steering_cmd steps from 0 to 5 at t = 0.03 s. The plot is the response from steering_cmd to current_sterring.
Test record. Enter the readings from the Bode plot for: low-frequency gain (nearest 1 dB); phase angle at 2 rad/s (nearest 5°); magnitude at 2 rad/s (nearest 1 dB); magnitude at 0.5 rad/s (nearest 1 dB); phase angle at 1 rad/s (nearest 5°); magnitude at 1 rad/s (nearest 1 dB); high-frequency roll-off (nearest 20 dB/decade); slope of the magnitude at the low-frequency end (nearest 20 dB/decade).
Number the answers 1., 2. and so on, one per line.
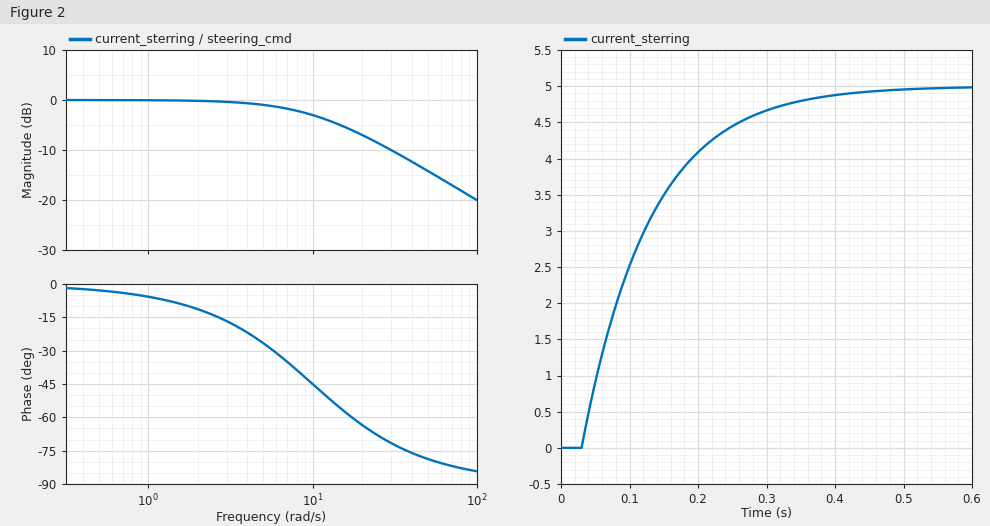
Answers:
1. 0 dB
2. -10°
3. 0 dB
4. 0 dB
5. -5°
6. 0 dB
7. -20 dB/decade
8. 0 dB/decade
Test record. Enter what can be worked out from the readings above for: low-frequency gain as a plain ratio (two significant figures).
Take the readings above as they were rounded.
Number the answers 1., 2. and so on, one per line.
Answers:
1. 1.0
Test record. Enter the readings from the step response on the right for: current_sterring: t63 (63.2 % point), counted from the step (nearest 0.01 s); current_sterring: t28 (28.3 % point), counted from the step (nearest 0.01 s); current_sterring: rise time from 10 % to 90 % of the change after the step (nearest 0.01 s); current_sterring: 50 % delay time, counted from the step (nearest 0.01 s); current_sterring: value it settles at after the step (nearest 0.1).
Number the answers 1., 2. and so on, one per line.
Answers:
1. 0.10 s
2. 0.03 s
3. 0.22 s
4. 0.07 s
5. 5.0
